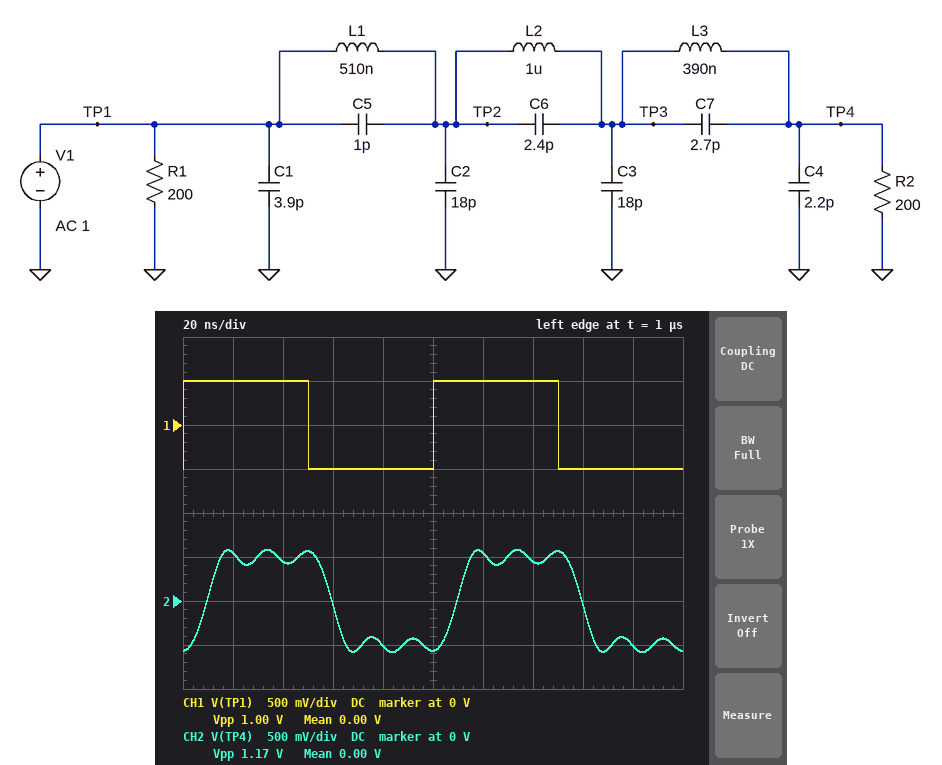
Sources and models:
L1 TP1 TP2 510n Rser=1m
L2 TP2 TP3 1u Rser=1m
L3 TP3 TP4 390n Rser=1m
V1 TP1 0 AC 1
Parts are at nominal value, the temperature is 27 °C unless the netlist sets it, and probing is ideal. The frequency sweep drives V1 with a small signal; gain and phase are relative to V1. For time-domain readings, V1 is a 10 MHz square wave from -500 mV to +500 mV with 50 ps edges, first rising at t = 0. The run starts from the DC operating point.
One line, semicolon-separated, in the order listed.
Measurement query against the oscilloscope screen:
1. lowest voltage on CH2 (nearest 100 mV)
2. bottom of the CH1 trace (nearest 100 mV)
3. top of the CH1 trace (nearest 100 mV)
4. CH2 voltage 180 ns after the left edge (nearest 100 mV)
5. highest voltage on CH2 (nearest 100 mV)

-600 mV; -500 mV; 500 mV; -500 mV; 600 mV
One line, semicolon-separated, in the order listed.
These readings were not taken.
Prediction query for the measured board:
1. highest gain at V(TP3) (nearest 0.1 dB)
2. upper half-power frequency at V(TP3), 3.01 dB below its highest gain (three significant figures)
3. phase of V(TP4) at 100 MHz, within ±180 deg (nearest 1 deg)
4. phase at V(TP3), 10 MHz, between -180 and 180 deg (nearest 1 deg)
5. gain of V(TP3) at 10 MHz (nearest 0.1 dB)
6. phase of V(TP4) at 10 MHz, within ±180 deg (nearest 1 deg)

11.2 dB; 62.6 MHz; -72 deg; -27 deg; -0.1 dB; -34 deg
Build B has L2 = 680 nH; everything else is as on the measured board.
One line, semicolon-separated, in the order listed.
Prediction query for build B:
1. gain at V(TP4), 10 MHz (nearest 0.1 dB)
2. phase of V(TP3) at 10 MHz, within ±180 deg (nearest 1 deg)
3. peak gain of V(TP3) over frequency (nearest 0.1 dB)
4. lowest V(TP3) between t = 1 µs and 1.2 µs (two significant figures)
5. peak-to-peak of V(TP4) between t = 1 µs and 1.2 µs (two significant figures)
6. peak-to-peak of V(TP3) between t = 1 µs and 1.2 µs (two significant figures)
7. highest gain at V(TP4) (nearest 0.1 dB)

0.1 dB; -22 deg; 7.4 dB; -850 mV; 1.6 V; 1.7 V; 5.0 dB
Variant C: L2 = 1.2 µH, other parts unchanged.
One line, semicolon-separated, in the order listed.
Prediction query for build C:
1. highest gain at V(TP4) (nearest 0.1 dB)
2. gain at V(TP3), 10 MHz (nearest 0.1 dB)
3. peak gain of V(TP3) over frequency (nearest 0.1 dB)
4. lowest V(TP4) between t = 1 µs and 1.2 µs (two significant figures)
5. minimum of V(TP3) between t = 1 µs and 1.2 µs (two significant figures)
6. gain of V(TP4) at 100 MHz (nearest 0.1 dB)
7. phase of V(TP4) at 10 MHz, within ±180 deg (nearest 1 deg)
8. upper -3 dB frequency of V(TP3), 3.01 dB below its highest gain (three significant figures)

11.7 dB; -0.3 dB; 13.3 dB; -570 mV; -590 mV; -52.0 dB; -37 deg; 59.7 MHz
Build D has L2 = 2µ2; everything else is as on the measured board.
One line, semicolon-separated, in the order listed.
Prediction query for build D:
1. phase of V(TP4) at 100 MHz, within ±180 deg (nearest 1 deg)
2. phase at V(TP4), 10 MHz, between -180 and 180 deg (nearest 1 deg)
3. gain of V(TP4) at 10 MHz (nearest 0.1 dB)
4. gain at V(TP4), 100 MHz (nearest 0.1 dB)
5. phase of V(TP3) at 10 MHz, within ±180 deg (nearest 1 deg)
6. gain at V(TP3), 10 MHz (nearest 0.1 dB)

108 deg; -51 deg; -1.6 dB; -40.4 dB; -44 deg; -1.5 dB
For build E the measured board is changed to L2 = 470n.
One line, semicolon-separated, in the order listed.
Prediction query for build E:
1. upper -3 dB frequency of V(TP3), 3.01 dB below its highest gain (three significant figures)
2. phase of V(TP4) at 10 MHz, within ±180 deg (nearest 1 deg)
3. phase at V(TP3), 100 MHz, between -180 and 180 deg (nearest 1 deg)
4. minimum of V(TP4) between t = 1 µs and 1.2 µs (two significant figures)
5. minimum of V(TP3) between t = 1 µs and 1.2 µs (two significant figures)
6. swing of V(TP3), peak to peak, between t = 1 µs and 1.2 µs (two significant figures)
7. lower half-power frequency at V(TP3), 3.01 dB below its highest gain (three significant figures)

81.9 MHz; -25 deg; 9 deg; -740 mV; -780 mV; 1.6 V; 74.0 MHz
